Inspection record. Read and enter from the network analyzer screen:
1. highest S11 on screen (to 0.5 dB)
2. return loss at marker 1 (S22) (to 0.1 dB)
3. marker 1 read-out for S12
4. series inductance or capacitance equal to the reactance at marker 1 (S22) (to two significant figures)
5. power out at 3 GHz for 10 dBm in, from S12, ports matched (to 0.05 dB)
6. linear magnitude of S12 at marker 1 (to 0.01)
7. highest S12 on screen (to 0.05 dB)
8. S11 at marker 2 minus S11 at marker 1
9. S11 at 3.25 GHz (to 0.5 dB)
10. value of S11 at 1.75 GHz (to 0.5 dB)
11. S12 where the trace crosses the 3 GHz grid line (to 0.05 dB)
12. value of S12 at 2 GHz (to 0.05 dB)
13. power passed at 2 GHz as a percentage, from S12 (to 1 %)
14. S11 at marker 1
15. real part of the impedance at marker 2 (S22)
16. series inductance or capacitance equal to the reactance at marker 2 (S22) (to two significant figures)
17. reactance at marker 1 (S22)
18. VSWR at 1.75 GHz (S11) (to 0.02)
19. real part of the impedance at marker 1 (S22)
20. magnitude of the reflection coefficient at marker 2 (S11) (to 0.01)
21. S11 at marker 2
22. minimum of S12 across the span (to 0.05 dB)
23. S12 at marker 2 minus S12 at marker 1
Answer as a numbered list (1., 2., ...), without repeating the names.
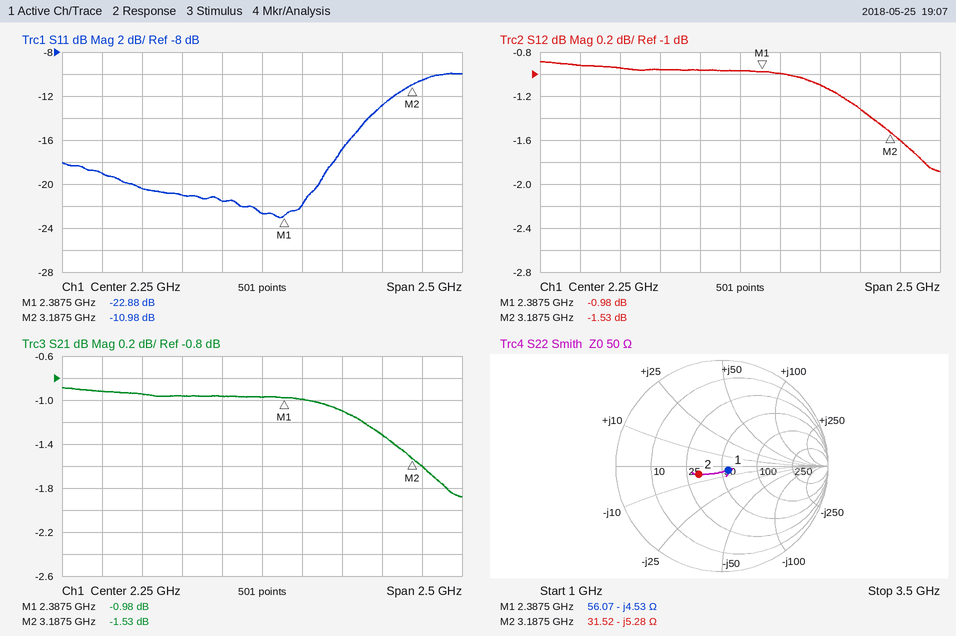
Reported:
1. -10.0 dB
2. 22.9 dB
3. -0.98 dB
4. 15 pF
5. 8.70 dBm
6. 0.89
7. -0.90 dB
8. 11.90 dB
9. -10.5 dB
10. -21.0 dB
11. -1.30 dB
12. -0.95 dB
13. 80 %
14. -22.88 dB
15. 31.52 Ω
16. 9.5 pF
17. -4.53 Ω
18. 1.20
19. 56.07 Ω
20. 0.28
21. -10.98 dB
22. -1.90 dB
23. -0.55 dB
